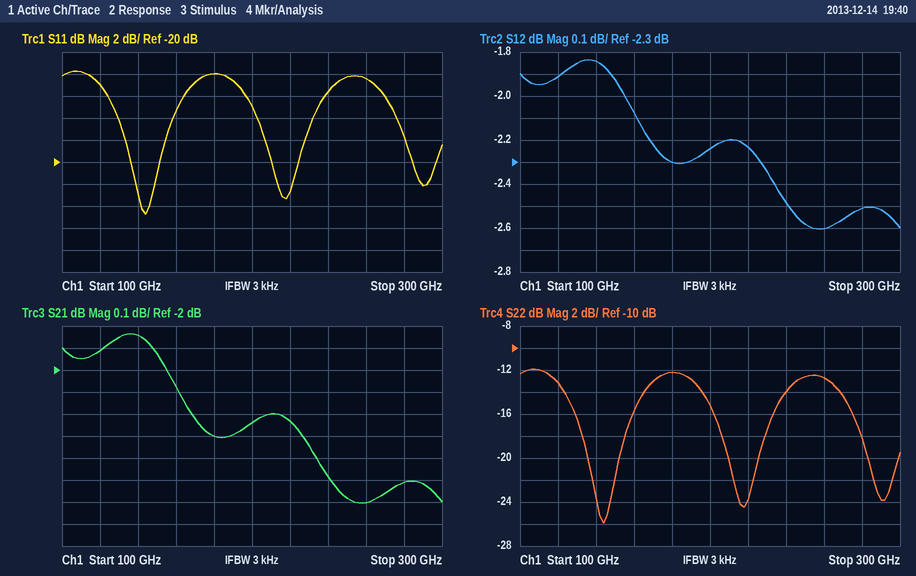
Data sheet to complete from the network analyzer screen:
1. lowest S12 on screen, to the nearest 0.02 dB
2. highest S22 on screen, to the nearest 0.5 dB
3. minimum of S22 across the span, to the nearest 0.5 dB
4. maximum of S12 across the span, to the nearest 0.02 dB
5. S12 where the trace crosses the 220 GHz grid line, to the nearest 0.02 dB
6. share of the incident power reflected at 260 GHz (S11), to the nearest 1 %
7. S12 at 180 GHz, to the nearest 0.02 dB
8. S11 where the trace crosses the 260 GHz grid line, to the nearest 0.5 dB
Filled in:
-2.60 dB
-12.0 dB
-26.0 dB
-1.84 dB
-2.24 dB
6 %
-2.30 dB
-12.5 dB
